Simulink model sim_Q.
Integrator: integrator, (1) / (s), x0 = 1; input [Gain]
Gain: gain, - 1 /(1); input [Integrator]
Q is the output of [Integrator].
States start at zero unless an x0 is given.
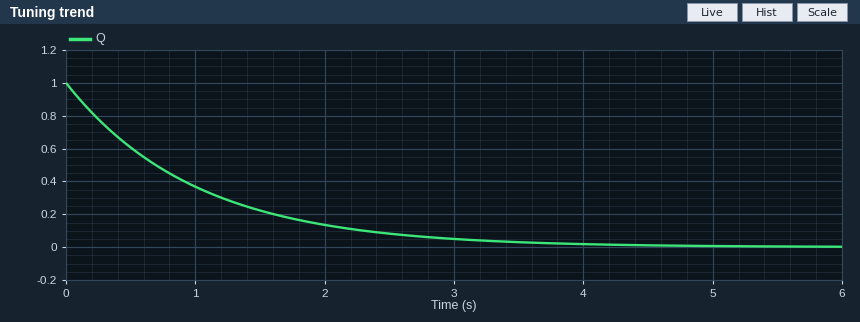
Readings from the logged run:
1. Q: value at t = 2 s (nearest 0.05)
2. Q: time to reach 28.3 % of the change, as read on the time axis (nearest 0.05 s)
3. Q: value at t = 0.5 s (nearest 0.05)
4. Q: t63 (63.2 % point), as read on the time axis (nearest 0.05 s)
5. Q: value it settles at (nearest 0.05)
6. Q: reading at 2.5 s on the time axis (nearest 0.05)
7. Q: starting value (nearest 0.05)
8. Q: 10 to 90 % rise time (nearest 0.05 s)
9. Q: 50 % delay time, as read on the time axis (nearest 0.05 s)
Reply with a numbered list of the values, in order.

1. 0.15
2. 0.35 s
3. 0.60
4. 1.00 s
5. 0.00
6. 0.10
7. 1.00
8. 2.20 s
9. 0.70 s
